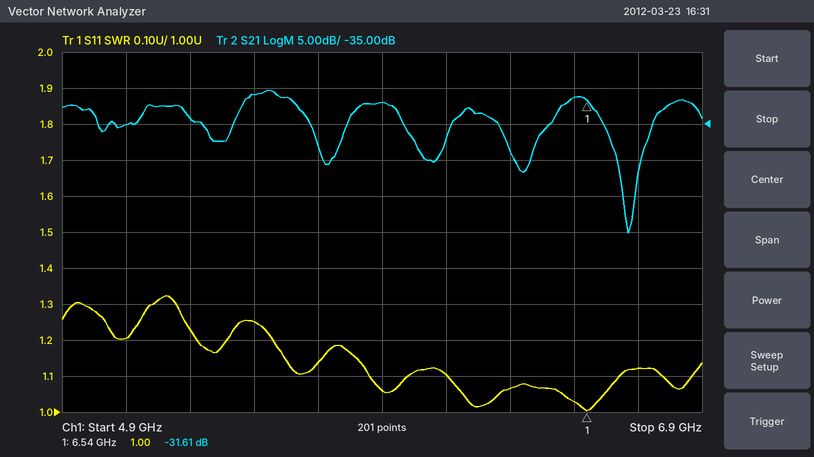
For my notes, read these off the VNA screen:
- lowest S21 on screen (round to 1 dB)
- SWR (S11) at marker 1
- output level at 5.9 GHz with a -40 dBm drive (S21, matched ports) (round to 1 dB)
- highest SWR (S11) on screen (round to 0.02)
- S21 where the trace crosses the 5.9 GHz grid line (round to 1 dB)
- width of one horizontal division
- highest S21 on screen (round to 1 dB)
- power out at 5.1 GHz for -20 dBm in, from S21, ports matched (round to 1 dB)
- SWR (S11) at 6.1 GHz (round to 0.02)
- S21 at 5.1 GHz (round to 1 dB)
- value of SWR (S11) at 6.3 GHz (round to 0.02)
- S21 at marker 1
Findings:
-50 dB
1.00
-72 dBm
1.32
-32 dB
200 MHz
-30 dB
-55 dBm
1.10
-35 dB
1.06
-31.61 dB
